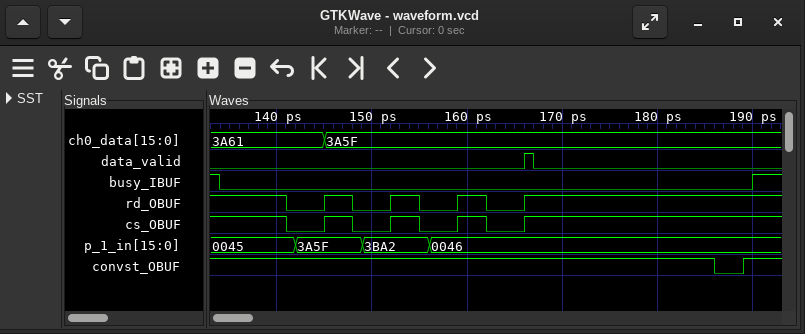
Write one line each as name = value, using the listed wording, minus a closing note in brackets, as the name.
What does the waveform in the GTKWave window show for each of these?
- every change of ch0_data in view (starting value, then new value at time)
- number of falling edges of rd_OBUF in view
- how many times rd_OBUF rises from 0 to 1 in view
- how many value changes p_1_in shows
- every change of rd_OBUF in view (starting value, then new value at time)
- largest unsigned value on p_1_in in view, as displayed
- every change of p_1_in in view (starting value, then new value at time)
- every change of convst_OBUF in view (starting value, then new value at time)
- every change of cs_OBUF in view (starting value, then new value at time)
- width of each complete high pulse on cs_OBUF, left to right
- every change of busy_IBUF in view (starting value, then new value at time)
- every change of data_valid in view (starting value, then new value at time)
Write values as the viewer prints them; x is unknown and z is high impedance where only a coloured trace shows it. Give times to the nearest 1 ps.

every change of ch0_data in view = 3A61, 3A5F at 145 ps
number of falling edges of rd_OBUF in view = 4
how many times rd_OBUF rises from 0 to 1 in view = 4
how many value changes p_1_in shows = 3
every change of rd_OBUF in view = 1, 0 at 141 ps, 1 at 145 ps, 0 at 148 ps, 1 at 152 ps, 0 at 155 ps, 1 at 159 ps, 0 at 162 ps, 1 at 166 ps
largest unsigned value on p_1_in in view, as displayed = 3BA2
every change of p_1_in in view = 0045, 3A5F at 142 ps, 3BA2 at 149 ps, 0046 at 156 ps
every change of convst_OBUF in view = 1, 0 at 186 ps, 1 at 189 ps
every change of cs_OBUF in view = 1, 0 at 141 ps, 1 at 145 ps, 0 at 148 ps, 1 at 152 ps, 0 at 155 ps, 1 at 159 ps, 0 at 162 ps, 1 at 166 ps
width of each complete high pulse on cs_OBUF, left to right = 3 ps, 3 ps, 3 ps
every change of busy_IBUF in view = 1, 0 at 134 ps, 1 at 190 ps
every change of data_valid in view = 0, 1 at 166 ps, 0 at 167 ps
